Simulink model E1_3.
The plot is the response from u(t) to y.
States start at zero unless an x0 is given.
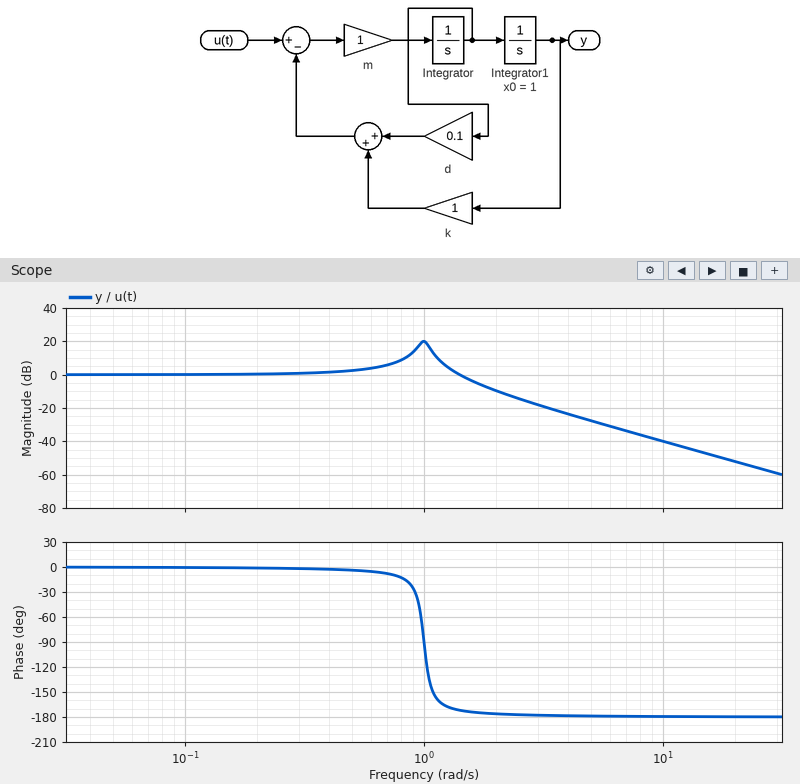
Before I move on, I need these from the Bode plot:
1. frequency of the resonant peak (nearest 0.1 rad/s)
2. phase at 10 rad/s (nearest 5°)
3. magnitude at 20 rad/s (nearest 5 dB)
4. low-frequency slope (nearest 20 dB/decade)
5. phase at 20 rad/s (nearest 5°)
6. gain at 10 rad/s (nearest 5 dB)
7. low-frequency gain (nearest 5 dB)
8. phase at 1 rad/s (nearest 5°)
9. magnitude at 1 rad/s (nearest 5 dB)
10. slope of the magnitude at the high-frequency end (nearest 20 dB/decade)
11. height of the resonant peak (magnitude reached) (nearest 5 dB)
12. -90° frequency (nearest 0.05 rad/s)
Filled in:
1.0 rad/s
-180°
-50 dB
0 dB/decade
-180°
-40 dB
0 dB
-90°
20 dB
-40 dB/decade
20 dB
1.00 rad/s
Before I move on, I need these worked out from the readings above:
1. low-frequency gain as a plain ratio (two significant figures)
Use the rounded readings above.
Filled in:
1.0
